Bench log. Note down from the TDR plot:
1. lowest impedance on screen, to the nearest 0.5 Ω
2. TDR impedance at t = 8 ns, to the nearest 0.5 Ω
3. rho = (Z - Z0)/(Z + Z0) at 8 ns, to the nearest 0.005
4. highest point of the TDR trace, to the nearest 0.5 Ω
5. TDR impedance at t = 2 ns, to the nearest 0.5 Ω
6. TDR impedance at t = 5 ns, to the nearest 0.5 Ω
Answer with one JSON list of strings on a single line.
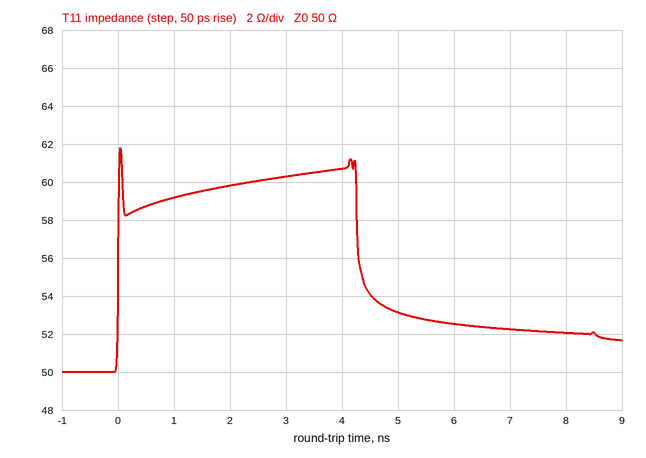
["50.0 Ω", "52.0 Ω", "+0.020", "62.0 Ω", "60.0 Ω", "53.0 Ω"]
